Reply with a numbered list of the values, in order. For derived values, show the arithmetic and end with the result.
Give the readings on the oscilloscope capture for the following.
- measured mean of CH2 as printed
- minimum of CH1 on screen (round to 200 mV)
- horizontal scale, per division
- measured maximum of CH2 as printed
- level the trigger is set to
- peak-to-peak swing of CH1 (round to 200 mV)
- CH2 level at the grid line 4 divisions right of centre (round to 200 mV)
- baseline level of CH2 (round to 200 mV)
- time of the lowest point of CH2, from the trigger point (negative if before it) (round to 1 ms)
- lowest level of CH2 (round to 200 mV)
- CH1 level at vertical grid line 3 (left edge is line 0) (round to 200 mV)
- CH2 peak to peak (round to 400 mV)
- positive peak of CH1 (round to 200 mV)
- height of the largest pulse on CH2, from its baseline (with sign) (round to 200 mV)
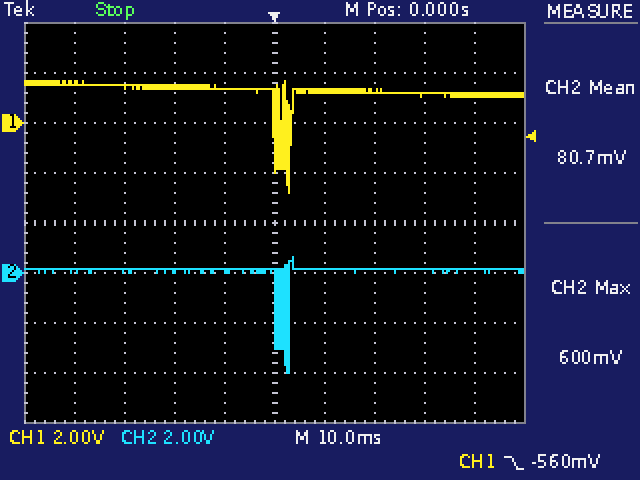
1. 80.7 mV
2. -2.8 V
3. 10 ms
4. 600 mV
5. -560 mV
6. 1.6 V − (-2.8 V) = 4.4 V
7. 200 mV
8. 200 mV
9. +3 ms
10. -4.0 V
11. 1.4 V
12. 4.8 V
13. 1.6 V
14. -4.0 V − (200 mV) = -4.2 V
